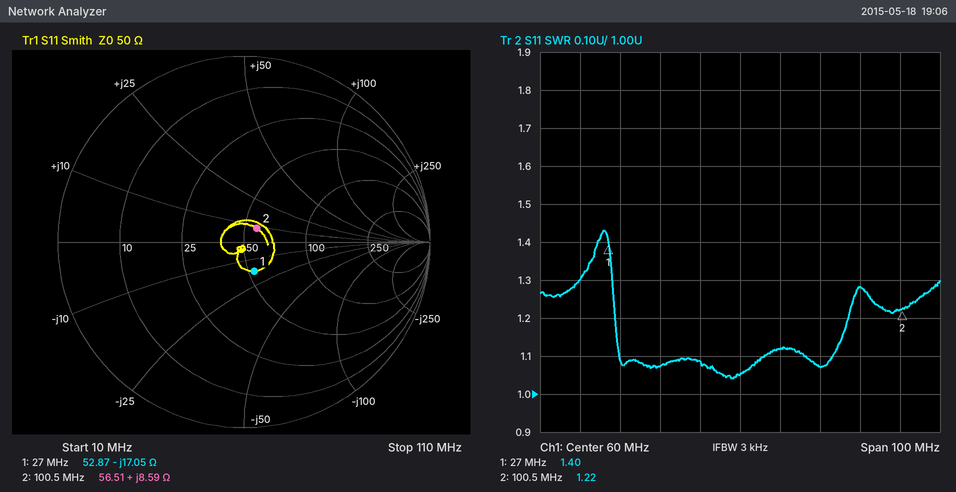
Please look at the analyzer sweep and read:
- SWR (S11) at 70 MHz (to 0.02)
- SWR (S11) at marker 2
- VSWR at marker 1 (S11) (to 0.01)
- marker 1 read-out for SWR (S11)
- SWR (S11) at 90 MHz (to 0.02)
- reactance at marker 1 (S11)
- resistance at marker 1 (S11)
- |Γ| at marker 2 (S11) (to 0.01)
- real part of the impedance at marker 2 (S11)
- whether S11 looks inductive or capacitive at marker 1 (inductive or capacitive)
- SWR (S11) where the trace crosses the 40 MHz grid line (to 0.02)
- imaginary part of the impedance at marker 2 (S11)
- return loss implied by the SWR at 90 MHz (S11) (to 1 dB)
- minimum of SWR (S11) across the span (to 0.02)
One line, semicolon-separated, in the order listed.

1.12; 1.22; 1.40; 1.40; 1.28; -17.05 Ω; 52.87 Ω; 0.10; 56.51 Ω; capacitive; 1.08; +8.59 Ω; 18 dB; 1.04
